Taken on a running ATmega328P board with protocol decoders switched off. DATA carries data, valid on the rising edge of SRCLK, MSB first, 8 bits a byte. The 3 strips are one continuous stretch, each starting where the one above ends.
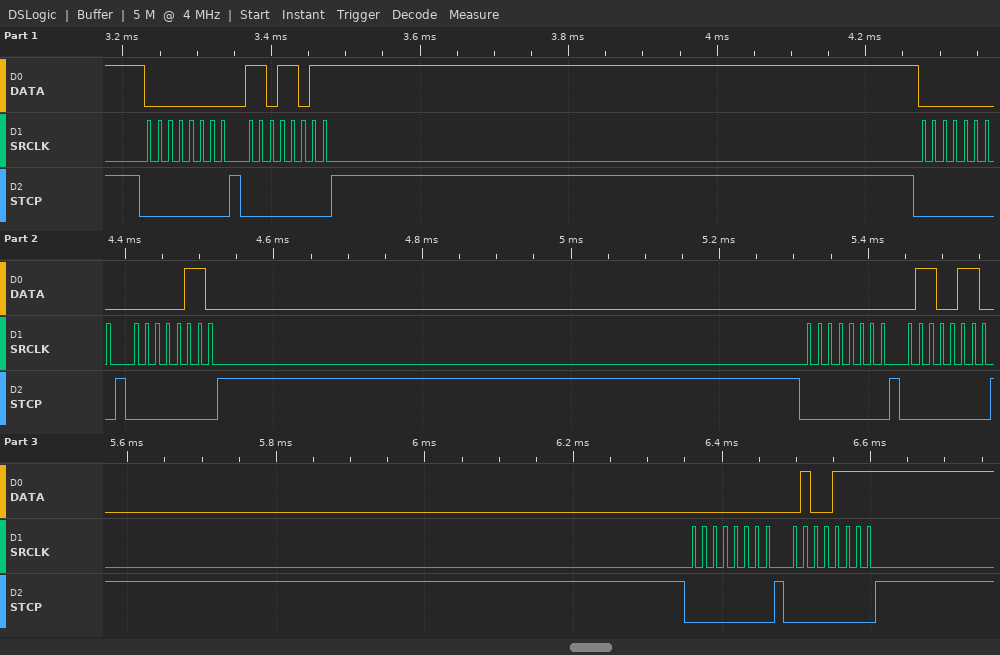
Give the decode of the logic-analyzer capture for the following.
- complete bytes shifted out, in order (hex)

00 DB 00 06 00 66 00 4F
